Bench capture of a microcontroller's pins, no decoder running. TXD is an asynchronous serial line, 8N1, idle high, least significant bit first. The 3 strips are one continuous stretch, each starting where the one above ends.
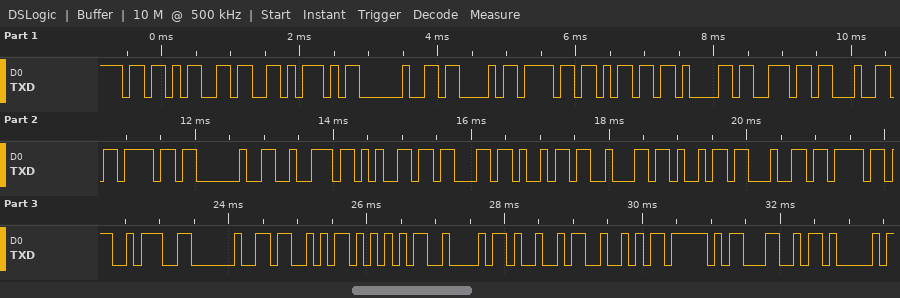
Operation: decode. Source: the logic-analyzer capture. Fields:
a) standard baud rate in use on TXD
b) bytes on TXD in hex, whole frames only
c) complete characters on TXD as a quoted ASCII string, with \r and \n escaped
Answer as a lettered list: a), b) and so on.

a) 9600 baud
b) 5B 36 5D 20 43 6F 6D 61 6E 64 6F 20 72 65 63 69 62 69 64 6F 3A 20 53 55 42 49 52 5F 4C 41
c) "[6] Comando recibido: SUBIR_LA"
